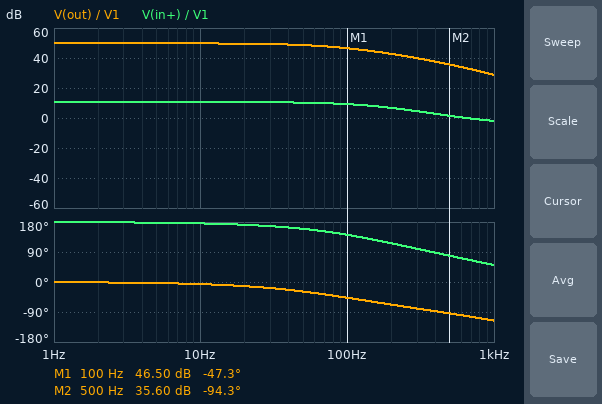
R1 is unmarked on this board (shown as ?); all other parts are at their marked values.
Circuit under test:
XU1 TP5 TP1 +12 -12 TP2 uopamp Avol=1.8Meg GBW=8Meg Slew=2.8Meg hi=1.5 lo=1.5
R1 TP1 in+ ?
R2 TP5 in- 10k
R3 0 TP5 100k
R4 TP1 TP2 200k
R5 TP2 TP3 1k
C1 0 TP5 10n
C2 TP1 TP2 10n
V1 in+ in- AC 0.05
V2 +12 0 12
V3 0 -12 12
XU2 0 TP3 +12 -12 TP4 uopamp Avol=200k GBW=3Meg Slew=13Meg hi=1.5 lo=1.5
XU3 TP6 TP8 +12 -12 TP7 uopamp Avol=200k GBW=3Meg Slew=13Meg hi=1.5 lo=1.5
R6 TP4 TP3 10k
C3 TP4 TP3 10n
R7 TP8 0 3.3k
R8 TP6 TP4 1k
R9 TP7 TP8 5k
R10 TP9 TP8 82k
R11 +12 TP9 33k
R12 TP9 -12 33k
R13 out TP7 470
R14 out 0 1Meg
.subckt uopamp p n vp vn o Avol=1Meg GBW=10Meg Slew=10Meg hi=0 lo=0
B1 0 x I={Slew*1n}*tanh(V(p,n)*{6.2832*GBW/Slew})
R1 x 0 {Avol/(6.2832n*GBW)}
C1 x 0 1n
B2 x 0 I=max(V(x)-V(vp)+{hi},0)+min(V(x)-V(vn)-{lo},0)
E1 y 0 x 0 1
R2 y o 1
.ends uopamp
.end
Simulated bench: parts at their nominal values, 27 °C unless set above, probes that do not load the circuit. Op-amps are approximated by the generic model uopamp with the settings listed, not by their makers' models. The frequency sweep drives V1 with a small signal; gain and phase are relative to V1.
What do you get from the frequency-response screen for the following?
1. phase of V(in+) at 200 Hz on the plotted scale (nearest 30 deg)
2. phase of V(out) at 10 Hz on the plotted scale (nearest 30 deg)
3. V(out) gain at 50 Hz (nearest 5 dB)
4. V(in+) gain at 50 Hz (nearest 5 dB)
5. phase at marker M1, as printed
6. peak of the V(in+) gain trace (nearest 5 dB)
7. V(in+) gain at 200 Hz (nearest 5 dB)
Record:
120 deg
0 deg
50 dB
10 dB
-47.3 deg
10 dB
5 dB
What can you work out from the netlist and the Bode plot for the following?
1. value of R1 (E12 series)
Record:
15 kΩ
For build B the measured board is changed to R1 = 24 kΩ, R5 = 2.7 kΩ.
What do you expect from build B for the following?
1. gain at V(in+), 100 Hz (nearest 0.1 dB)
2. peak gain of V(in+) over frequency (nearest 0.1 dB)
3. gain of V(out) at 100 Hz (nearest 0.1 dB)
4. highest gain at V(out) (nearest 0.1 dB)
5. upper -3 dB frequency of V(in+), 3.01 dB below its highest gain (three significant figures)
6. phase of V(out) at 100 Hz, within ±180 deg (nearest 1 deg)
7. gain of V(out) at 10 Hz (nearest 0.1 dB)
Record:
5.7 dB
7.0 dB
35.2 dB
38.5 dB
178 Hz
-47 deg
38.4 dB
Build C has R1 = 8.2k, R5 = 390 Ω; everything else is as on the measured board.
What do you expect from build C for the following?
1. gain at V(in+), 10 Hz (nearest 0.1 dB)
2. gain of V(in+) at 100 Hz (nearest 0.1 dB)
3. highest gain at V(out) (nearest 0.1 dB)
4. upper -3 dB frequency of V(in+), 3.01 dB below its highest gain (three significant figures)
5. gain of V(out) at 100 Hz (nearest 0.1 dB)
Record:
14.0 dB
12.6 dB
60.7 dB
160 Hz
57.4 dB
